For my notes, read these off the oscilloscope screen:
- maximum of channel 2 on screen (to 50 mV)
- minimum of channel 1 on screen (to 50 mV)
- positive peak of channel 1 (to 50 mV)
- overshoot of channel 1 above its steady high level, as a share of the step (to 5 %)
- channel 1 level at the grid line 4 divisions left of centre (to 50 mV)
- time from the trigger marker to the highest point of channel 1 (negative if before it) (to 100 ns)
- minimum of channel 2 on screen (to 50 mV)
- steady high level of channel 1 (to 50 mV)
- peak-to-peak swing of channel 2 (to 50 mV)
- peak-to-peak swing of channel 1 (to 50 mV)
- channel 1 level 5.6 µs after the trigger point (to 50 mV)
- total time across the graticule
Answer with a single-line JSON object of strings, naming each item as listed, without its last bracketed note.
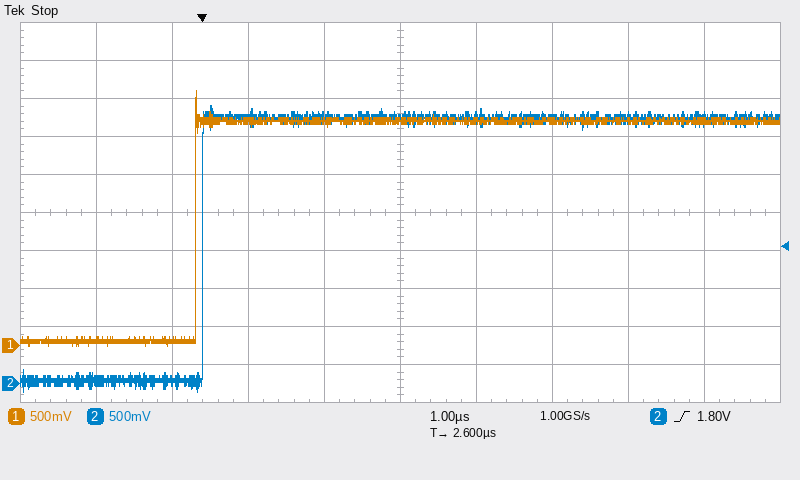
{"maximum of channel 2 on screen": "3.65 V", "minimum of channel 1 on screen": "0 mV", "positive peak of channel 1": "3.35 V", "overshoot of channel 1 above its steady high level, as a share of the step": "15 %", "channel 1 level at the grid line 4 divisions left of centre": "100 mV", "time from the trigger marker to the highest point of channel 1 (negative if before it)": "-100 ns", "minimum of channel 2 on screen": "-100 mV", "steady high level of channel 1": "2.95 V", "peak-to-peak swing of channel 2": "3.75 V", "peak-to-peak swing of channel 1": "3.35 V", "channel 1 level 5.6 µs after the trigger point": "2.95 V", "total time across the graticule": "10 µs"}
